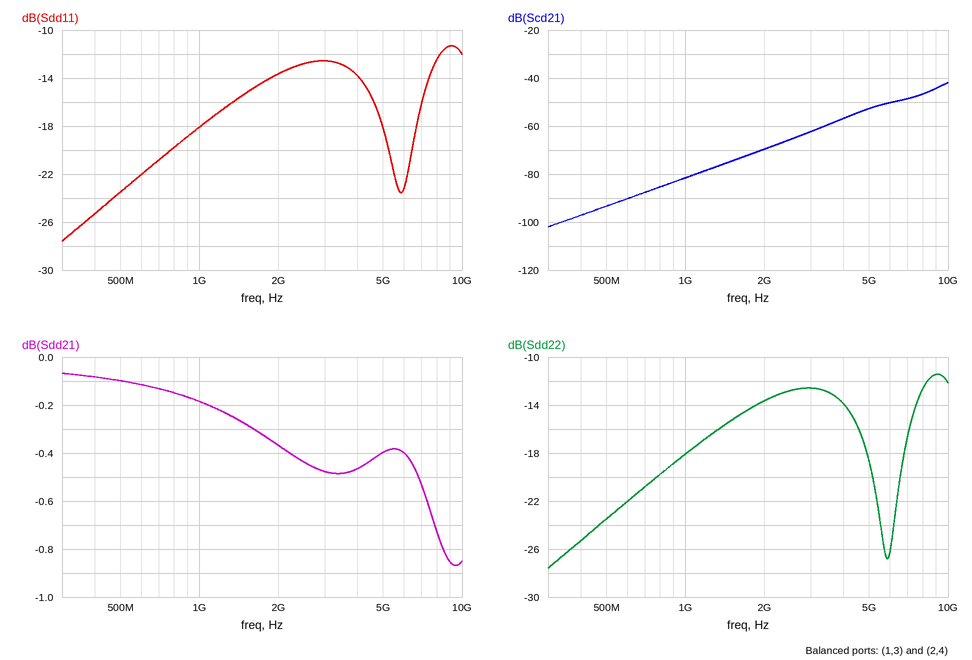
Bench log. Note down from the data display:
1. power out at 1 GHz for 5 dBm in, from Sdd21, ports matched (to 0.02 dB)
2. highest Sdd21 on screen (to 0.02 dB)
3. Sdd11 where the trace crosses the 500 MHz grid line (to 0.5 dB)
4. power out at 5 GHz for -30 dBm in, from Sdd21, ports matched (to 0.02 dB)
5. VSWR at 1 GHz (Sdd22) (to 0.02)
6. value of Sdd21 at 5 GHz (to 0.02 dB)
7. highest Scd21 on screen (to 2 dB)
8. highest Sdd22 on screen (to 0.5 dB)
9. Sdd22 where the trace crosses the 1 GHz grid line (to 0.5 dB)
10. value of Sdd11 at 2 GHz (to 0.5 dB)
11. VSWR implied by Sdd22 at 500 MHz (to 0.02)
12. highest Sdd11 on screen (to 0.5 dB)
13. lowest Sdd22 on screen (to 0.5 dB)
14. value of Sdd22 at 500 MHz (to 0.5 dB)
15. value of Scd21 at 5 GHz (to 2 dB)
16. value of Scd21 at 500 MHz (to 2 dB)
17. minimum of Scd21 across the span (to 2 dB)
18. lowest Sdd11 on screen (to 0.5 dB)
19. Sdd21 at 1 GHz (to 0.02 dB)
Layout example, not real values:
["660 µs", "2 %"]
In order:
["4.82 dBm", "-0.06 dB", "-23.5 dB", "-30.40 dBm", "1.28", "-0.40 dB", "-42 dB", "-11.5 dB", "-18.0 dB", "-13.5 dB", "1.14", "-11.5 dB", "-27.5 dB", "-23.5 dB", "-52 dB", "-94 dB", "-102 dB", "-27.5 dB", "-0.18 dB"]
